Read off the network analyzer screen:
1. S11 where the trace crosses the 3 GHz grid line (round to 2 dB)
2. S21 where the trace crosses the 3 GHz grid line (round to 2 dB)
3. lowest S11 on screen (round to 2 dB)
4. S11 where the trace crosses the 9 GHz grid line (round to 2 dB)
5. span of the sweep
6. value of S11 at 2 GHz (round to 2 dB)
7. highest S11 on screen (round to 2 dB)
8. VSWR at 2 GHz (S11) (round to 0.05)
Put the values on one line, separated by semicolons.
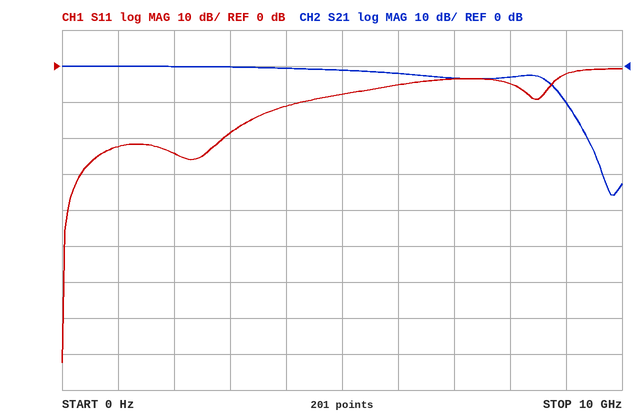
-18 dB; 0 dB; -82 dB; -2 dB; 10 GHz; -24 dB; 0 dB; 1.15
